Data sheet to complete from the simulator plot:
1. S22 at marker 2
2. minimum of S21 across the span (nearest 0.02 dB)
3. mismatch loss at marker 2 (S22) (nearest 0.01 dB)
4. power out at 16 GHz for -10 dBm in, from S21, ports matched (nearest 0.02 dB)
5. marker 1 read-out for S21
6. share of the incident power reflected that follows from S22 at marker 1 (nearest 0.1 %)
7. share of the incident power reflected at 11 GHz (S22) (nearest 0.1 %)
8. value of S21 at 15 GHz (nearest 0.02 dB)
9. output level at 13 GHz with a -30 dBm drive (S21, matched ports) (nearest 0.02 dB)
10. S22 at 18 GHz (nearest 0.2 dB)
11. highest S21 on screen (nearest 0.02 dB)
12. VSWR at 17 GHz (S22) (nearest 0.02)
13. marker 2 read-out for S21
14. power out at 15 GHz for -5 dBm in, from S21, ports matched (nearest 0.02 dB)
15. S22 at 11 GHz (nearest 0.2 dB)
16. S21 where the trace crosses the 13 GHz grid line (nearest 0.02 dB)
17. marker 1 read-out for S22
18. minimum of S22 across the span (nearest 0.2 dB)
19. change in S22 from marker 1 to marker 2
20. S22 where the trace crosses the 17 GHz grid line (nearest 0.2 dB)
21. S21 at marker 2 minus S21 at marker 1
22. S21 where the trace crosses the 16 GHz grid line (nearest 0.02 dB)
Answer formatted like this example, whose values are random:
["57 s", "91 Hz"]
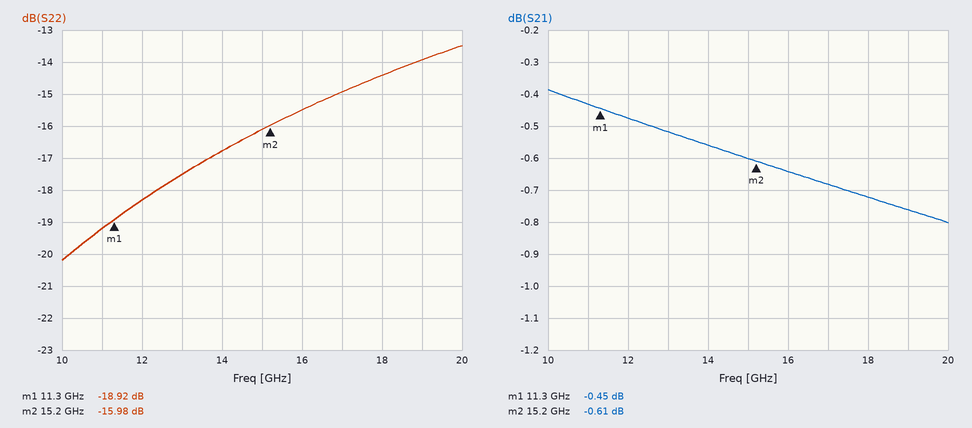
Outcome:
["-15.98 dB", "-0.80 dB", "0.11 dB", "-10.64 dBm", "-0.45 dB", "1.3 %", "1.2 %", "-0.60 dB", "-30.52 dBm", "-14.4 dB", "-0.38 dB", "1.44", "-0.61 dB", "-5.60 dBm", "-19.2 dB", "-0.52 dB", "-18.92 dB", "-20.2 dB", "2.94 dB", "-15.0 dB", "-0.16 dB", "-0.64 dB"]
